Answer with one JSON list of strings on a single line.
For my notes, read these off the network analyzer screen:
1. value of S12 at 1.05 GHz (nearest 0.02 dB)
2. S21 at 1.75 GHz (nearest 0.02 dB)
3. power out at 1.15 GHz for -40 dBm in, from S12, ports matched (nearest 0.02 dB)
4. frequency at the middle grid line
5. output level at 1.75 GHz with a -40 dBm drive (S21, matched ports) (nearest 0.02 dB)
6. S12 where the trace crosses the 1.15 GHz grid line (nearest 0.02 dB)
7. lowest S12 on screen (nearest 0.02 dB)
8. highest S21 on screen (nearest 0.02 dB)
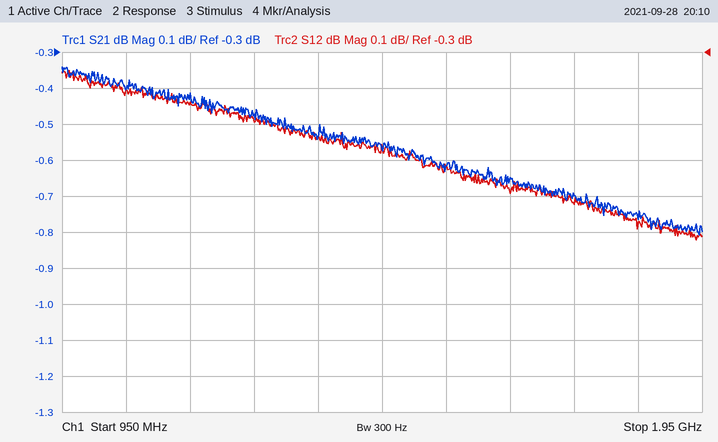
["-0.40 dB", "-0.70 dB", "-40.44 dBm", "1.45 GHz", "-40.70 dBm", "-0.44 dB", "-0.82 dB", "-0.34 dB"]
